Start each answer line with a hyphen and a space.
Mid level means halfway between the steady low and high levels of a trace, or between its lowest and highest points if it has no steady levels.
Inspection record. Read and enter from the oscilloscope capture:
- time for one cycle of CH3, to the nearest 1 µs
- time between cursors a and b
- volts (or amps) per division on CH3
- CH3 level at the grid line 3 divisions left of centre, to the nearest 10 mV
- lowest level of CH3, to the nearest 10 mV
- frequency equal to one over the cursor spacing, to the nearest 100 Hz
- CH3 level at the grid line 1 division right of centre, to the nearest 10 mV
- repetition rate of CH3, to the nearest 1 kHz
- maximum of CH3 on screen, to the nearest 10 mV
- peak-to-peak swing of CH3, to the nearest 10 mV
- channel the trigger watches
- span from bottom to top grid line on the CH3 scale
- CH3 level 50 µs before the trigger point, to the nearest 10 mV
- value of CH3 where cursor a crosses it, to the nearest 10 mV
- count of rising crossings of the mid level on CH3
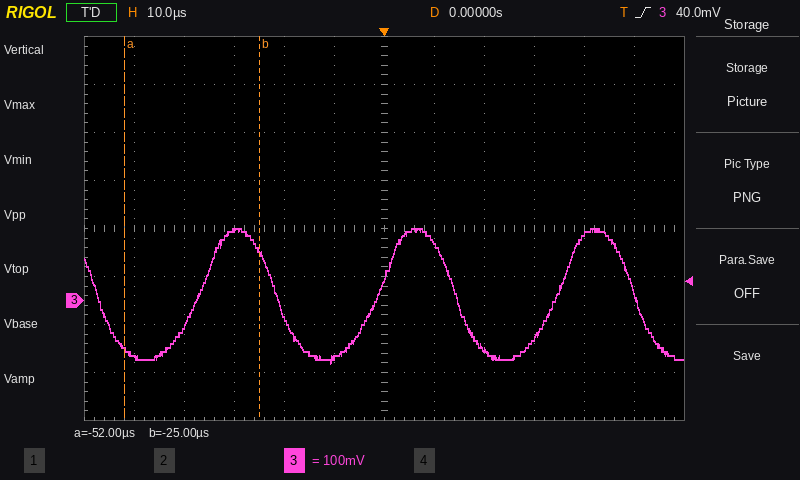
- 36 µs
- 27 µs
- 100 mV
- 150 mV
- -130 mV
- 37.0 kHz
- 120 mV
- 28 kHz
- 150 mV
- 280 mV
- CH3
- 800 mV
- -120 mV
- -100 mV
- 3
